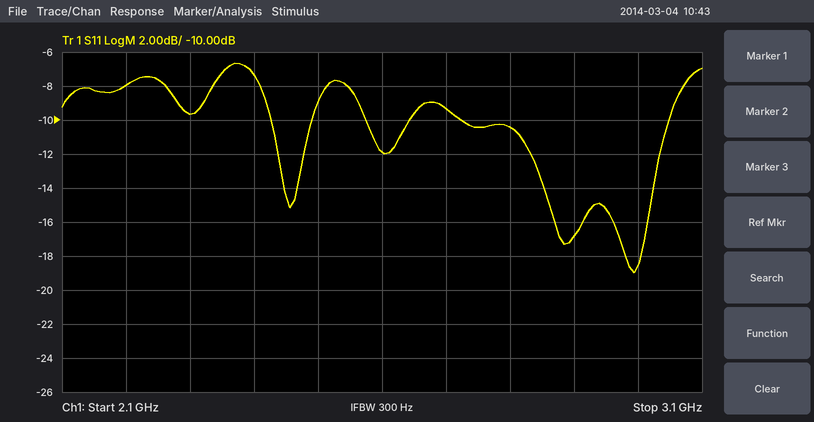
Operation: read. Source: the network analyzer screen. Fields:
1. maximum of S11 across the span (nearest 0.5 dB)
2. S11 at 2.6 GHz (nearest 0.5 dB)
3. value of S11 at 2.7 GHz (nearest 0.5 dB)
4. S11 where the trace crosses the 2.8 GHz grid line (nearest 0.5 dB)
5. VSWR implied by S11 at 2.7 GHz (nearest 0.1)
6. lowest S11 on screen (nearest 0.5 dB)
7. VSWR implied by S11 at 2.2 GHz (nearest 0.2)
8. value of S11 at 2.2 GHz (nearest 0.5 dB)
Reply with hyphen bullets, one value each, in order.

- -6.5 dB
- -12.0 dB
- -9.5 dB
- -10.5 dB
- 2.0
- -19.0 dB
- 2.4
- -8.0 dB
